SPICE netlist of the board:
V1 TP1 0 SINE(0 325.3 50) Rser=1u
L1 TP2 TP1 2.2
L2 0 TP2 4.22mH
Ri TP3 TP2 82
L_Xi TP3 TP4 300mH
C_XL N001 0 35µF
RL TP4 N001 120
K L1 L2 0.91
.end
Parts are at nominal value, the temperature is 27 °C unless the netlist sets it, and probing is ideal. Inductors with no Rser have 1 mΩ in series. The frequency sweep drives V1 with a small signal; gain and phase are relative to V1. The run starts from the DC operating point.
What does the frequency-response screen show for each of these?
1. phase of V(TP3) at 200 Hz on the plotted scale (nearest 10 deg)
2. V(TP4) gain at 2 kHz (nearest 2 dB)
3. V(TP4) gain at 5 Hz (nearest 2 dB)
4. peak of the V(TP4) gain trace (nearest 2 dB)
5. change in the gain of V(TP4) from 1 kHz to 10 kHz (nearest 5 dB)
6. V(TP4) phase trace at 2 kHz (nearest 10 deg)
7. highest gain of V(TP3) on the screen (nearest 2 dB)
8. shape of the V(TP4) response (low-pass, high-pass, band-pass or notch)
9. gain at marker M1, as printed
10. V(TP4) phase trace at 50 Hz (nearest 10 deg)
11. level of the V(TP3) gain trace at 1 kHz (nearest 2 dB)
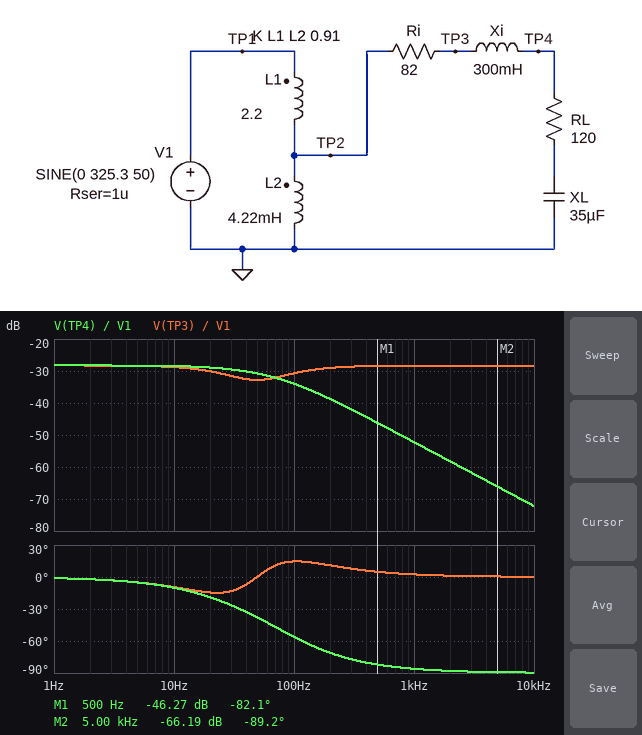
10 deg
-58 dB
-28 dB
-28 dB
-20 dB
-90 deg
-28 dB
low-pass
-46.27 dB
-40 deg
-28 dB
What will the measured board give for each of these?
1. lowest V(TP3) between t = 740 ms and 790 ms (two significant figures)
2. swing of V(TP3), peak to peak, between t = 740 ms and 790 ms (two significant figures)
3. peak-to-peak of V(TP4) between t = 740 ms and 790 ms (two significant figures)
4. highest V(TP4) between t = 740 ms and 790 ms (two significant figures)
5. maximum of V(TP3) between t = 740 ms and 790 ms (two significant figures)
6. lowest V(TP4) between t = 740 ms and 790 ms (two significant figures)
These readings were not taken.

-7.5 V
15 V
19 V
9.4 V
7.5 V
-9.4 V
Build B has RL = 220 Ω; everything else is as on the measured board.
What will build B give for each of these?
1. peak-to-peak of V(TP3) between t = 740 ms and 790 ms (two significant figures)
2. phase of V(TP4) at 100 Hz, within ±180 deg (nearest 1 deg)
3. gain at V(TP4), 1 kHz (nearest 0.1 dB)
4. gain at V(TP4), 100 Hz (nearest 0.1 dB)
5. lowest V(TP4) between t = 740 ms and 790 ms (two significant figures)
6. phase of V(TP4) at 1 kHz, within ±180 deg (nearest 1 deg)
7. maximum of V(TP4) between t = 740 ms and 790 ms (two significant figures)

18 V
-37 deg
-47.0 dB
-31.7 dB
-9.9 V
-82 deg
9.9 V
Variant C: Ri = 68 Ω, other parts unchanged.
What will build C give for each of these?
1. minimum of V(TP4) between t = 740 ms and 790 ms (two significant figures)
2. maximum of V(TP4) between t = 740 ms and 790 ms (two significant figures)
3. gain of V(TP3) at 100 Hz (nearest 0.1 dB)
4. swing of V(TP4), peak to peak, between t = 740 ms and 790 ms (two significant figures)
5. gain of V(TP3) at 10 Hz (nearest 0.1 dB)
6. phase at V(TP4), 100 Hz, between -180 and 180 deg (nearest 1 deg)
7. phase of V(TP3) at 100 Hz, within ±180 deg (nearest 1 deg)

-10 V
10 V
-30.3 dB
20 V
-28.7 dB
-58 deg
13 deg
